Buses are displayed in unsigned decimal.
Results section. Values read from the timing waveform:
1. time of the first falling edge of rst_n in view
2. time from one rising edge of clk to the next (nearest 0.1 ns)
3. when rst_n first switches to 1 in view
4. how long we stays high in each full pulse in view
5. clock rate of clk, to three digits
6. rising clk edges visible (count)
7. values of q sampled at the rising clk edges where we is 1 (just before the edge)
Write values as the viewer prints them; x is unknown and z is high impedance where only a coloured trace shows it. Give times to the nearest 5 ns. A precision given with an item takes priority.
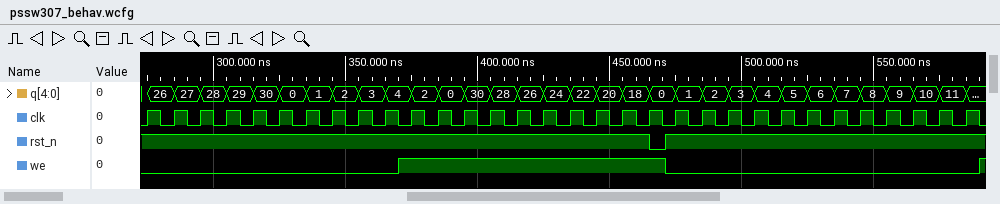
465 ns
10 ns
470 ns
100 ns
100 MHz
32
4, 2, 0, 30, 28, 26, 24, 22, 20, 18
